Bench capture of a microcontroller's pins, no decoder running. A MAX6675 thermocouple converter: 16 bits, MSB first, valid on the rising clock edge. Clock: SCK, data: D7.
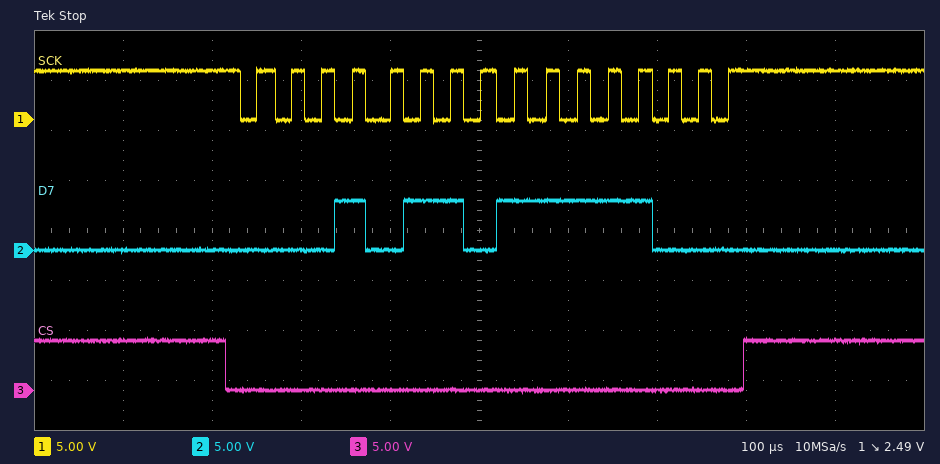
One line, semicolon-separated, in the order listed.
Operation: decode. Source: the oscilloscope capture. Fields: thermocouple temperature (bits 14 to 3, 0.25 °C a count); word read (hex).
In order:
183.75 °C; 0x16F8
